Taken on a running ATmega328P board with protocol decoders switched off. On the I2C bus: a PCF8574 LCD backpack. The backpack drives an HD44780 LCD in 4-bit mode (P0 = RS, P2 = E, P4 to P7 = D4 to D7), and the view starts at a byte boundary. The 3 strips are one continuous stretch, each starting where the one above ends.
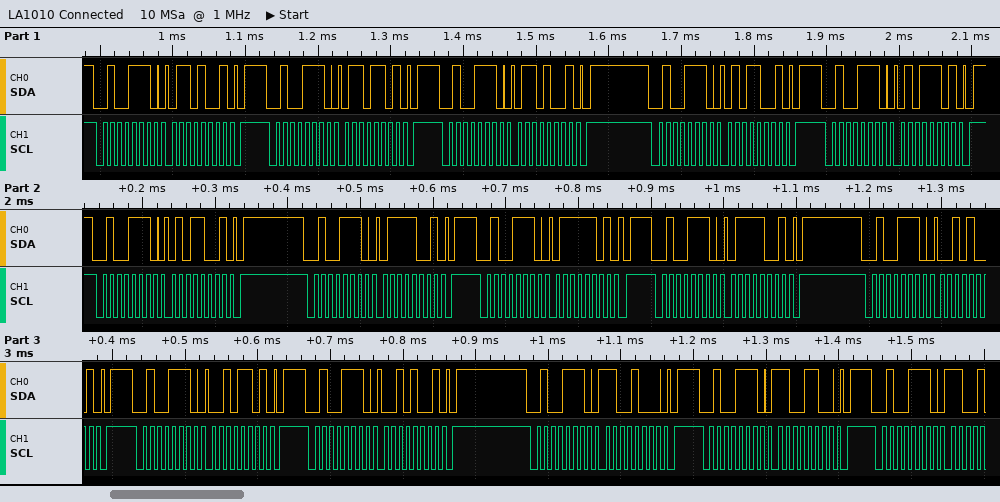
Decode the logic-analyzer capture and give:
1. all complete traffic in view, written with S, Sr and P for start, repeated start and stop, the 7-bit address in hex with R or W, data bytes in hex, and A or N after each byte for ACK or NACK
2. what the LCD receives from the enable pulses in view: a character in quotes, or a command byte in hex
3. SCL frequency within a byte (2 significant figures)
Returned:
S 27W A 69 A P S 27W A 6D A P S 27W A 69 A P S 27W A 59 A P S 27W A 5D A P S 27W A 59 A P S 27W A 79 A P S 27W A 7D A P S 27W A 79 A P S 27W A 29 A P S 27W A 2D A P S 27W A 29 A P S 27W A C8 A P S 27W A CC A P S 27W A
'e' 'r'
100 kHz
